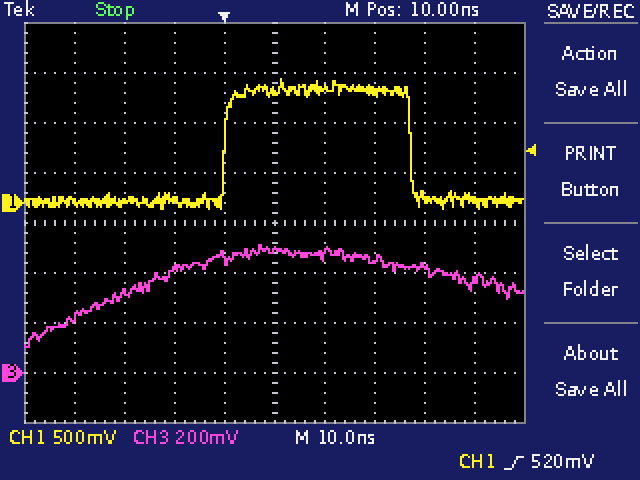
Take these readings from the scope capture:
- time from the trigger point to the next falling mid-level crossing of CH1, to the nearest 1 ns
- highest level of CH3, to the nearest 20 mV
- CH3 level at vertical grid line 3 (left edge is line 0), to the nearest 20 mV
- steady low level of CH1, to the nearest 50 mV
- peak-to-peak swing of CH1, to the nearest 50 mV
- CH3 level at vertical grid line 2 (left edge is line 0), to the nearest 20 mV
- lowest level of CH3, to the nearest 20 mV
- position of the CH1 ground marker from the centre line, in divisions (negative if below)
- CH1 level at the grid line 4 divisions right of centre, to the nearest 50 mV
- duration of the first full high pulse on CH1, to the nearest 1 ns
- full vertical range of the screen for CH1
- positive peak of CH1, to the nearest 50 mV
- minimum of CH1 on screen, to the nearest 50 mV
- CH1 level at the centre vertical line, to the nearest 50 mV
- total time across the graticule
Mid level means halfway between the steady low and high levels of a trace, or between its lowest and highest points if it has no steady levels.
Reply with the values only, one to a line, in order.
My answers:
37 ns
520 mV
420 mV
0 mV
1.30 V
320 mV
100 mV
+0.4 div
0 mV
37 ns
4 V
1.25 V
-50 mV
1.10 V
100 ns
